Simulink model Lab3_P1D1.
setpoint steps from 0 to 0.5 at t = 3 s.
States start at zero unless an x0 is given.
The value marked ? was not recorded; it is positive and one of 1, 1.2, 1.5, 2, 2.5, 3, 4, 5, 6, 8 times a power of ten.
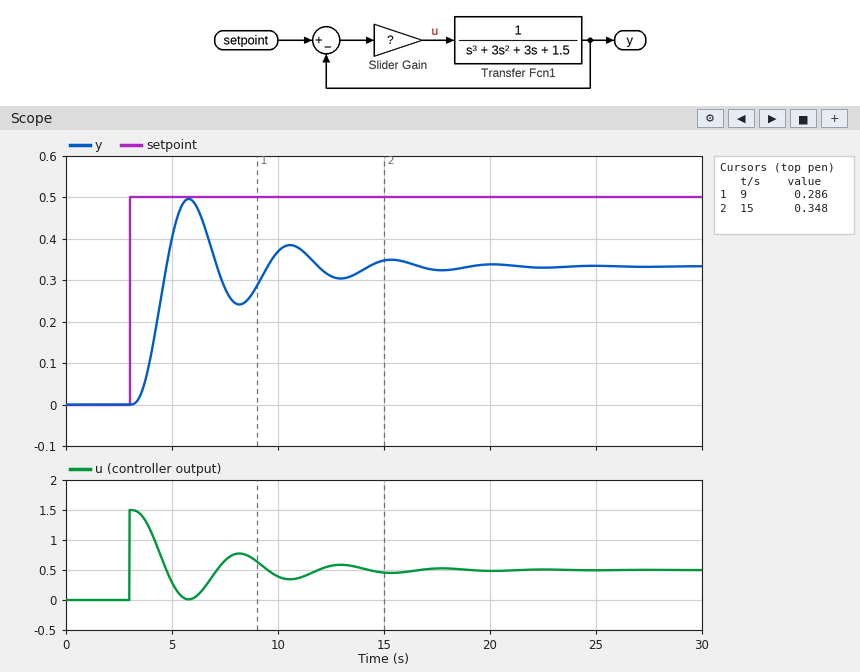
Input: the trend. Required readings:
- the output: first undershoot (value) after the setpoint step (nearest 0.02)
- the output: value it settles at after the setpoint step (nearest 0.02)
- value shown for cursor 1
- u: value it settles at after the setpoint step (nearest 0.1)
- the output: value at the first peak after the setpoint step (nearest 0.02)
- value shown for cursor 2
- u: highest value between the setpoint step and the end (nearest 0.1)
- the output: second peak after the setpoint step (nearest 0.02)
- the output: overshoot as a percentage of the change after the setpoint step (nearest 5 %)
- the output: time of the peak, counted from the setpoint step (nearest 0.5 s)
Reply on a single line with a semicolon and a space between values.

0.24; 0.34; 0.286; 0.5; 0.50; 0.348; 1.5; 0.38; 50 %; 3.0 s
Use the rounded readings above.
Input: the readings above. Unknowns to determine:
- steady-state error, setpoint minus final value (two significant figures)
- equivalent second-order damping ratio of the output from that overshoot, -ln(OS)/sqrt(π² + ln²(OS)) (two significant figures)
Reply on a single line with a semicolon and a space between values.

0.16; 0.22
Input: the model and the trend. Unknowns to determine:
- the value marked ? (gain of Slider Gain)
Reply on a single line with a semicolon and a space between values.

3
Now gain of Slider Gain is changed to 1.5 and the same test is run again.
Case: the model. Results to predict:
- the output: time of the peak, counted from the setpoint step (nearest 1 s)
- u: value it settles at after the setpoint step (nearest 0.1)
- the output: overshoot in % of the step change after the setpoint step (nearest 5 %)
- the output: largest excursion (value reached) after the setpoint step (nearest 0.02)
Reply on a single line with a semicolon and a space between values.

3 s; 0.4; 30 %; 0.32
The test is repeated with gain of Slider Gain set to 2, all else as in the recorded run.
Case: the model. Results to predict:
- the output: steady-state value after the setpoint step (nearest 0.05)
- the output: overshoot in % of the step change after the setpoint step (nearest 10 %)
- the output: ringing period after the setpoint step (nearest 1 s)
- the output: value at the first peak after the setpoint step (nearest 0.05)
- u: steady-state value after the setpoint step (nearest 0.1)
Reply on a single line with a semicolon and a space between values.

0.30; 40 %; 5 s; 0.40; 0.4
